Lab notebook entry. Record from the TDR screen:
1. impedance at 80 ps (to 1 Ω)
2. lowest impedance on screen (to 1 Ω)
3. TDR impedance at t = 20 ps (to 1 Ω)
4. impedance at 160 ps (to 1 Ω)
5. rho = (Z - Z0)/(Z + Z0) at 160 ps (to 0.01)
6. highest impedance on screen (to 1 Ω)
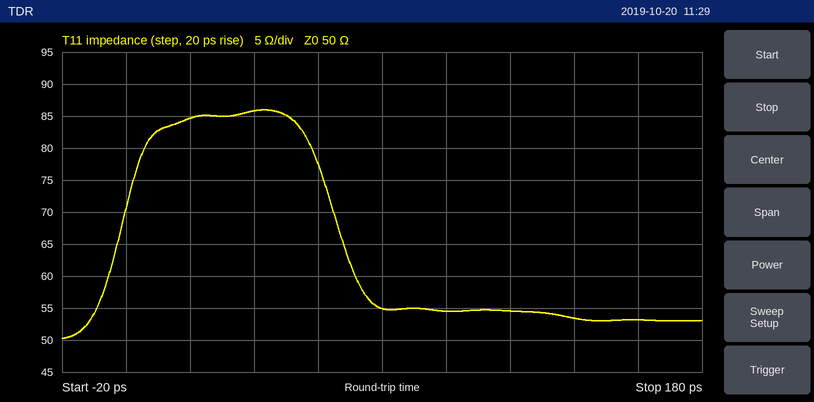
55 Ω
50 Ω
85 Ω
53 Ω
+0.03
86 Ω
